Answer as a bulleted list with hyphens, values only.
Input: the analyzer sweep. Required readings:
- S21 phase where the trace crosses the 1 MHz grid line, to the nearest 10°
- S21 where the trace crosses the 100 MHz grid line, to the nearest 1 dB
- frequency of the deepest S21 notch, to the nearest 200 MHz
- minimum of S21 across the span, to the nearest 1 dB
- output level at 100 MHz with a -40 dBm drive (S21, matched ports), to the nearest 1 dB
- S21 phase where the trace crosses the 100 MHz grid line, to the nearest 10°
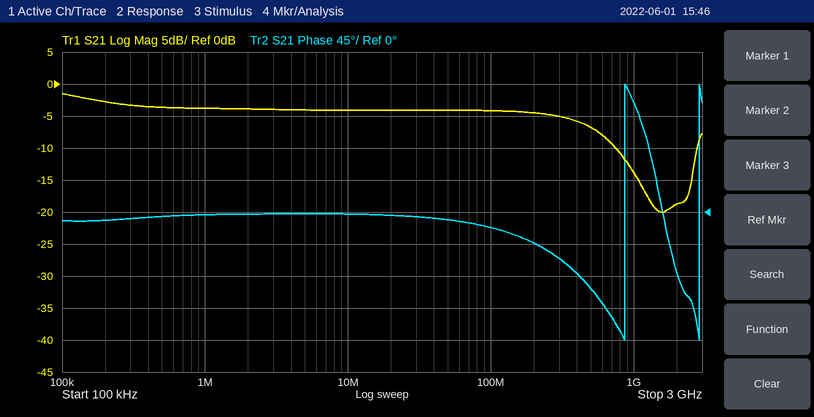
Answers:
- 0°
- -4 dB
- 1.6 GHz
- -20 dB
- -44 dBm
- -20°
